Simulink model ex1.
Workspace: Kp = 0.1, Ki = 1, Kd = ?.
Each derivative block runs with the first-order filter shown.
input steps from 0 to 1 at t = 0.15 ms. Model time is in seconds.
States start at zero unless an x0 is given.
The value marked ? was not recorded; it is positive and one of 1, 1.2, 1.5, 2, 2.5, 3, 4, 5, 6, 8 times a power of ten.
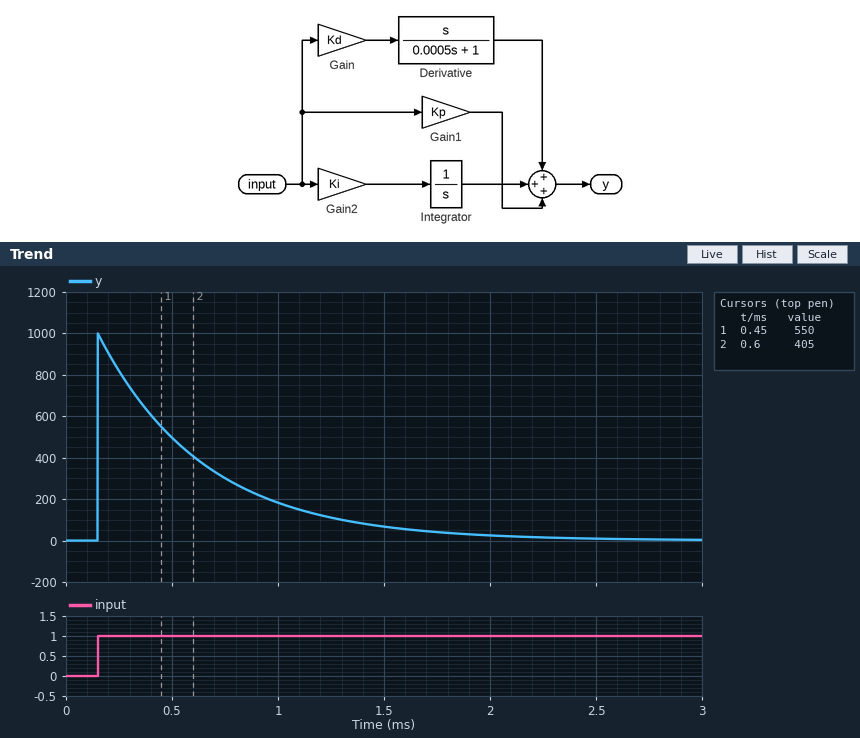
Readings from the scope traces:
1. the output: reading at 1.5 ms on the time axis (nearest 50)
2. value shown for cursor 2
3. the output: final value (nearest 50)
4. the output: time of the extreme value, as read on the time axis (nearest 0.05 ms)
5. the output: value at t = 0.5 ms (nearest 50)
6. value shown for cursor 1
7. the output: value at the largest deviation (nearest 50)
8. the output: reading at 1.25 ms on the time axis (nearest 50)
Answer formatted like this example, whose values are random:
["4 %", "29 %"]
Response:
["50", "405", "0", "0.15 ms", "500", "550", "1000", "100"]
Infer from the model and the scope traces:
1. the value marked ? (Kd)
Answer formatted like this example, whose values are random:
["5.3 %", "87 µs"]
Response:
["0.5"]
